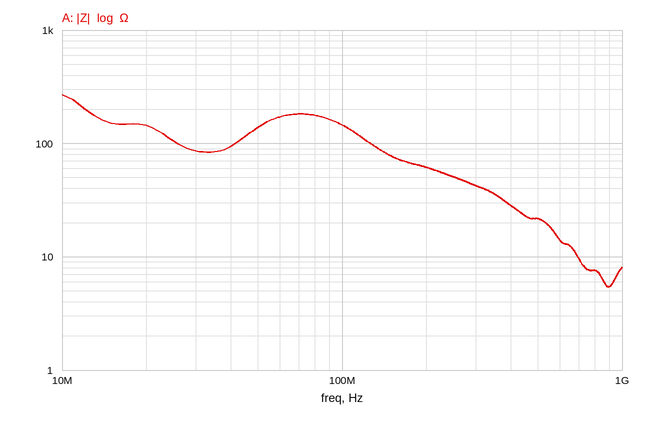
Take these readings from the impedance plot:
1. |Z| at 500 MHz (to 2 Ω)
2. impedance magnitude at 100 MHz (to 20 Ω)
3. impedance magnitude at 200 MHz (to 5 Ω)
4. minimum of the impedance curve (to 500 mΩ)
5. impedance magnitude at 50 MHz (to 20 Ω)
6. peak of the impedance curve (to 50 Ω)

22 Ω
140 Ω
60 Ω
5.5 Ω
140 Ω
250 Ω
